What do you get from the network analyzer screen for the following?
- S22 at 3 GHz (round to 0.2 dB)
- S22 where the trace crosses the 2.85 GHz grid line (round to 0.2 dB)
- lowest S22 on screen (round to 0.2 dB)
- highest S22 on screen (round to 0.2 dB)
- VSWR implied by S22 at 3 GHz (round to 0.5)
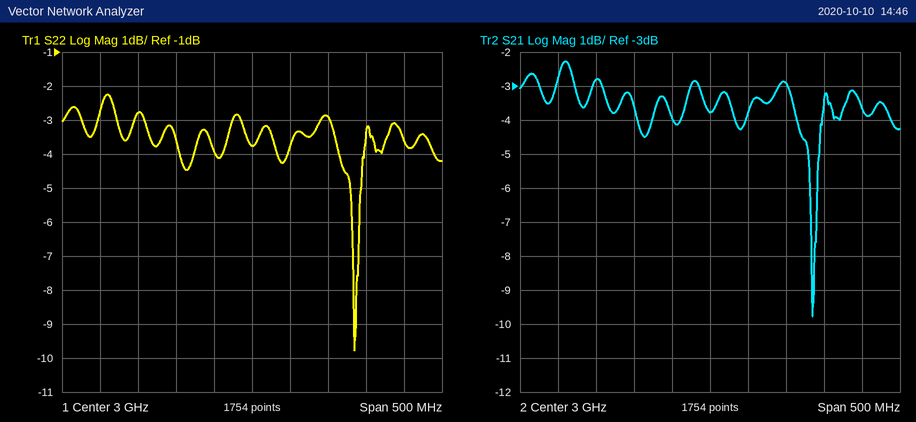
-3.8 dB
-2.8 dB
-9.8 dB
-2.2 dB
4.5
